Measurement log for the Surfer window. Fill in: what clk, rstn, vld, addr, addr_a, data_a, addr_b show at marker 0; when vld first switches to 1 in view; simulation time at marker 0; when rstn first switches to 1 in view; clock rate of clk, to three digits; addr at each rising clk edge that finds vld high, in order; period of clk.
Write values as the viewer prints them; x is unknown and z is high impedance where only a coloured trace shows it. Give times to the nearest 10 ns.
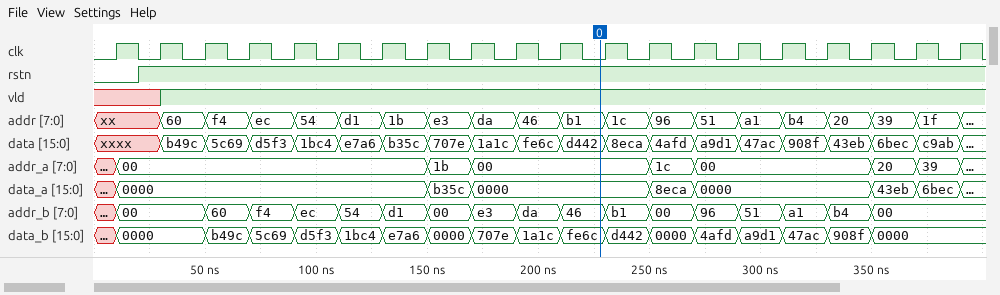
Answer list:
clk=0, rstn=1, vld=1, addr=b1, addr_a=00, data_a=0000, addr_b=46
30 ns
230 ns
20 ns
50.0 MHz
60, f4, ec, 54, d1, 1b, e3, da, 46, b1, 1c, 96, 51, a1, b4, 20, 39, 1f
20 ns
